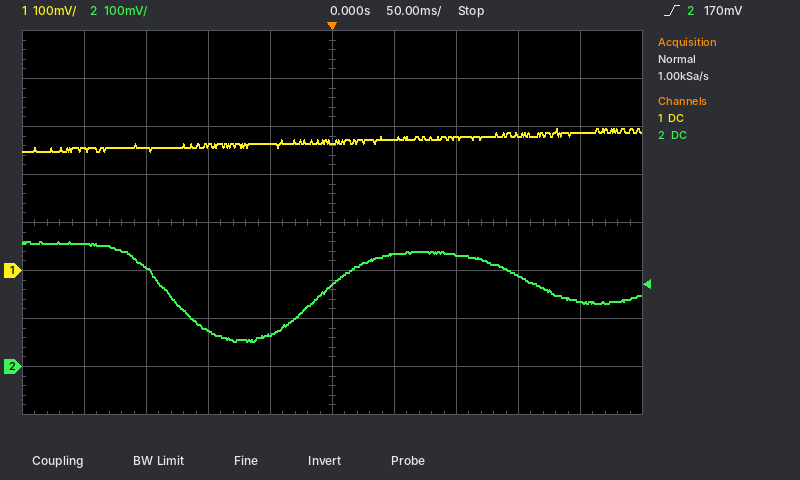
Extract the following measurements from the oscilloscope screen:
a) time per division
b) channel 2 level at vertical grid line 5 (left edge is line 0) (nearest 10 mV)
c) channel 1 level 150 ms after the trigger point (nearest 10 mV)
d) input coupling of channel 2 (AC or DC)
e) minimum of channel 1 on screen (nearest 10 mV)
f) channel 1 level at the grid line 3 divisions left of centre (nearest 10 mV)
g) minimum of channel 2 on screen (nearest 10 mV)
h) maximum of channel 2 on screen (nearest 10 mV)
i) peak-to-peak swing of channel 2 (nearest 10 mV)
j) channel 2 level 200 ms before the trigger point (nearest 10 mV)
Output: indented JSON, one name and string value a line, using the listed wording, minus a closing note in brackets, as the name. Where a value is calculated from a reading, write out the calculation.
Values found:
{
  "time per division": "50 ms",
  "channel 2 level at vertical grid line 5 (left edge is line 0)": "170 mV",
  "channel 1 level 150 ms after the trigger point": "280 mV",
  "input coupling of channel 2": "DC",
  "minimum of channel 1 on screen": "250 mV",
  "channel 1 level at the grid line 3 divisions left of centre": "260 mV",
  "minimum of channel 2 on screen": "50 mV",
  "maximum of channel 2 on screen": "260 mV",
  "peak-to-peak swing of channel 2": "260 mV − (50 mV) = 210 mV",
  "channel 2 level 200 ms before the trigger point": "260 mV"
}
